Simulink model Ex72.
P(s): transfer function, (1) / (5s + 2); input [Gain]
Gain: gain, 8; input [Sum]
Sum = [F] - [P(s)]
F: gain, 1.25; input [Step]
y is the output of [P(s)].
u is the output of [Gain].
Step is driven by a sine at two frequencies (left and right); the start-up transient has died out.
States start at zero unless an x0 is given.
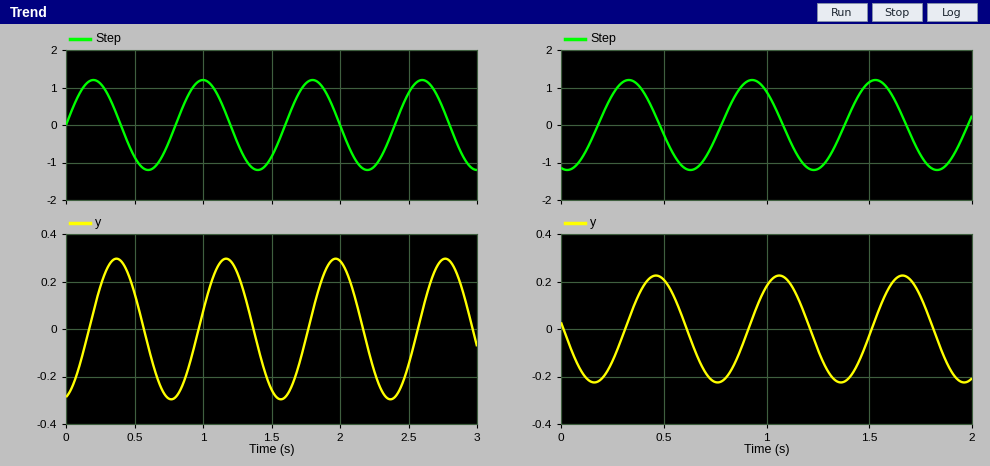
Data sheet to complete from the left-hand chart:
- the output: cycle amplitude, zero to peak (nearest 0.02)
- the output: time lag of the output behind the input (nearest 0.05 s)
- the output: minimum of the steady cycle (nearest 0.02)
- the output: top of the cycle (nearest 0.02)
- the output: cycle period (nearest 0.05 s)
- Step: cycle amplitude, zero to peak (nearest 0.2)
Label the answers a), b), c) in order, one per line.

a) 0.30
b) 0.15 s
c) -0.30
d) 0.30
e) 0.80 s
f) 1.2
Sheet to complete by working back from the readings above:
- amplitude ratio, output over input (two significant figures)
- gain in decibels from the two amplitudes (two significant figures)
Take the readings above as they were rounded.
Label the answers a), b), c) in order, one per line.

a) 0.25
b) -12 dB
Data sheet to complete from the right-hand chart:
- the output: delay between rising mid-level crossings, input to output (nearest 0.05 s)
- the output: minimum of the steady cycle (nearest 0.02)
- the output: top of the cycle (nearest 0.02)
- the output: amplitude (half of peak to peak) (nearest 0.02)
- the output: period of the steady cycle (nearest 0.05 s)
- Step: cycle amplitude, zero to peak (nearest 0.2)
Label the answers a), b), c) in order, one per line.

a) 0.15 s
b) -0.22
c) 0.22
d) 0.22
e) 0.60 s
f) 1.2
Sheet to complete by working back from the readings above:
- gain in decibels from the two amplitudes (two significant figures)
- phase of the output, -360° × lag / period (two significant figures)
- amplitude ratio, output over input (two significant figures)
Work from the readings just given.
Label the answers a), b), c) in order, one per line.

a) -15 dB
b) -90°
c) 0.18
